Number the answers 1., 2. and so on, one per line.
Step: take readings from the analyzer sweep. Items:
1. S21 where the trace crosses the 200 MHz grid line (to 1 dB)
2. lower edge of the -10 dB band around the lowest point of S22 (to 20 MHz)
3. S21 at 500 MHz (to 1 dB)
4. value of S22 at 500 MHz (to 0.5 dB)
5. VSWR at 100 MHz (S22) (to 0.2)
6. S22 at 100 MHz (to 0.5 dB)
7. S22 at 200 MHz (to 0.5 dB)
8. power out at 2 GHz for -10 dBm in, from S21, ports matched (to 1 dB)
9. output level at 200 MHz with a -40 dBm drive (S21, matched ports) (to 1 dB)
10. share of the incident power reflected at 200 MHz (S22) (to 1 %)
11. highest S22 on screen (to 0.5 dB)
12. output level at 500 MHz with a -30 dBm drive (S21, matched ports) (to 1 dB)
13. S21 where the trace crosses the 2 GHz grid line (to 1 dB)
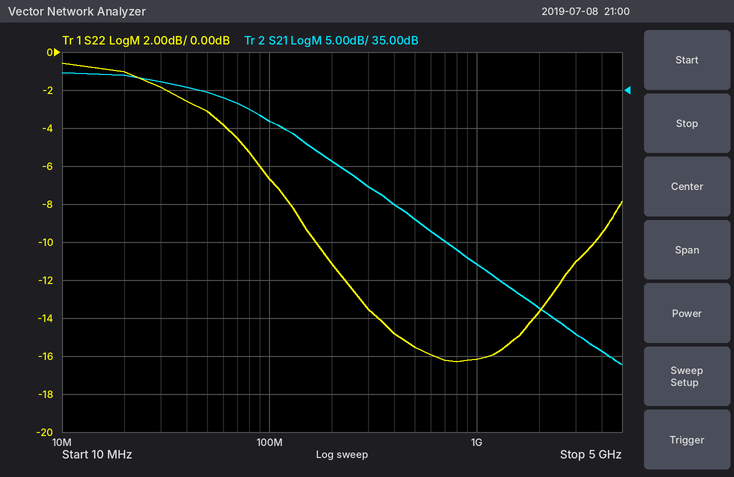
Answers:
1. 26 dB
2. 160 MHz
3. 18 dB
4. -15.5 dB
5. 2.8
6. -6.5 dB
7. -11.0 dB
8. -4 dBm
9. -14 dBm
10. 8 %
11. -0.5 dB
12. -12 dBm
13. 6 dB
